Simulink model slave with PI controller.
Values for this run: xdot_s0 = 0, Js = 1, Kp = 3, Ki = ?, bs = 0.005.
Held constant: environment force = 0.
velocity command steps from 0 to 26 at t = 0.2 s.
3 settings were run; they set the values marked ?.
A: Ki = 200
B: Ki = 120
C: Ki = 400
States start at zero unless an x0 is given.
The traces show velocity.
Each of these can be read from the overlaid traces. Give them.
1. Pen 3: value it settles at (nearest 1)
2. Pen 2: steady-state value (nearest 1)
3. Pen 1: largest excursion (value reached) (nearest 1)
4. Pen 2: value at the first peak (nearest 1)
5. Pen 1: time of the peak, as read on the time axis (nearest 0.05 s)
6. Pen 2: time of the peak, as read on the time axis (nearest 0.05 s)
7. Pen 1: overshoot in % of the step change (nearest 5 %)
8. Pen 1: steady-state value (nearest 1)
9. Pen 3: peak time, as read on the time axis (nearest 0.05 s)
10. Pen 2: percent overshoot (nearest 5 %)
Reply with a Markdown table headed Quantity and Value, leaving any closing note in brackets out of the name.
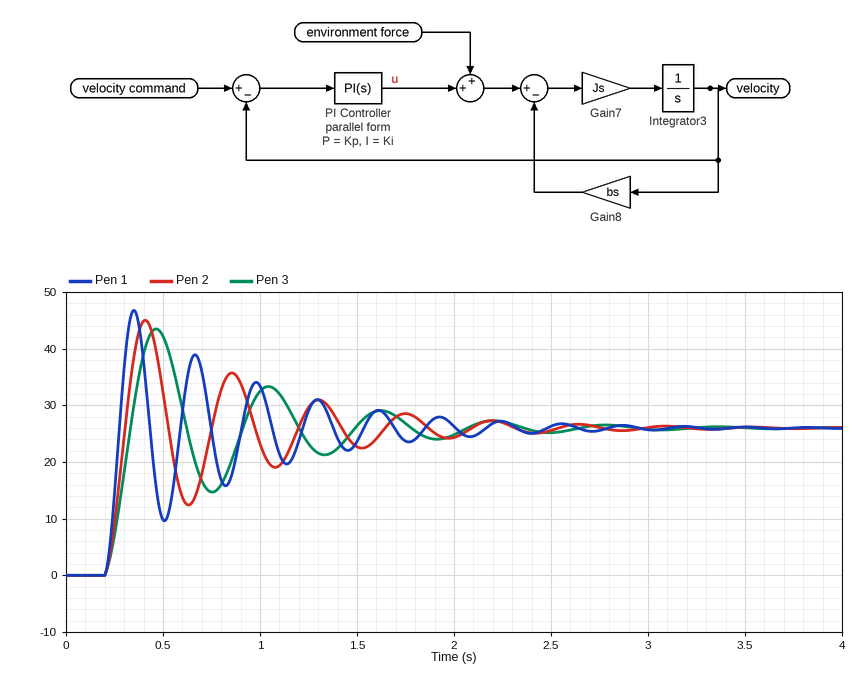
| Quantity | Value |
|---|---|
| Pen 3: value it settles at | 26 |
| Pen 2: steady-state value | 26 |
| Pen 1: largest excursion (value reached) | 47 |
| Pen 2: value at the first peak | 45 |
| Pen 1: time of the peak, as read on the time axis | 0.35 s |
| Pen 2: time of the peak, as read on the time axis | 0.40 s |
| Pen 1: overshoot in % of the step change | 80 % |
| Pen 1: steady-state value | 26 |
| Pen 3: peak time, as read on the time axis | 0.45 s |
| Pen 2: percent overshoot | 75 % |
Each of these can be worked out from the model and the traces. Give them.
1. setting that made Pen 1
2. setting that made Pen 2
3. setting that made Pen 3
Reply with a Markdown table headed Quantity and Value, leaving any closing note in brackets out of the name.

| Quantity | Value |
|---|---|
| setting that made Pen 1 | C |
| setting that made Pen 2 | A |
| setting that made Pen 3 | B |
